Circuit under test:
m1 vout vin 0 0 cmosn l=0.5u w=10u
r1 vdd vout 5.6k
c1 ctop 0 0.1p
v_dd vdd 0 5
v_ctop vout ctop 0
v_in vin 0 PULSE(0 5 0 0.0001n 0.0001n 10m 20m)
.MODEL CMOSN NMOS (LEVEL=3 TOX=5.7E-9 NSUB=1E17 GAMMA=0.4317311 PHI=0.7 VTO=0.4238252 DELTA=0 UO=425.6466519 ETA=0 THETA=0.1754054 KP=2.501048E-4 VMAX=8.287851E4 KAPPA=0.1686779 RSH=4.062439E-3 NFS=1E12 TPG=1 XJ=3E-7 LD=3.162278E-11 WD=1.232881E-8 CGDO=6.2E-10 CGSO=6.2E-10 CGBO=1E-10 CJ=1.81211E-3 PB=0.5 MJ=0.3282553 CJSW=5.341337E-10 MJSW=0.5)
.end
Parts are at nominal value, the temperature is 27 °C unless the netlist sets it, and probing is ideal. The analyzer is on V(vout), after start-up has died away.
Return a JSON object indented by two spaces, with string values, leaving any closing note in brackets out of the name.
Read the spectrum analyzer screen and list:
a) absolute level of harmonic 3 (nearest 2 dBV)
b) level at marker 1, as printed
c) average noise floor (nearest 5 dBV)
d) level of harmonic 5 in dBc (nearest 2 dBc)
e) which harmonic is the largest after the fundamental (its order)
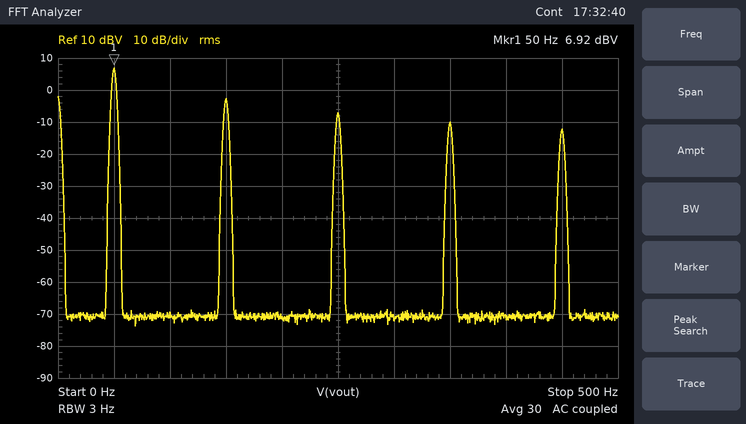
{
  "absolute level of harmonic 3": "-2 dBV",
  "level at marker 1, as printed": "6.92 dBV",
  "average noise floor": "-70 dBV",
  "level of harmonic 5 in dBc": "-14 dBc",
  "which harmonic is the largest after the fundamental": "3"
}
